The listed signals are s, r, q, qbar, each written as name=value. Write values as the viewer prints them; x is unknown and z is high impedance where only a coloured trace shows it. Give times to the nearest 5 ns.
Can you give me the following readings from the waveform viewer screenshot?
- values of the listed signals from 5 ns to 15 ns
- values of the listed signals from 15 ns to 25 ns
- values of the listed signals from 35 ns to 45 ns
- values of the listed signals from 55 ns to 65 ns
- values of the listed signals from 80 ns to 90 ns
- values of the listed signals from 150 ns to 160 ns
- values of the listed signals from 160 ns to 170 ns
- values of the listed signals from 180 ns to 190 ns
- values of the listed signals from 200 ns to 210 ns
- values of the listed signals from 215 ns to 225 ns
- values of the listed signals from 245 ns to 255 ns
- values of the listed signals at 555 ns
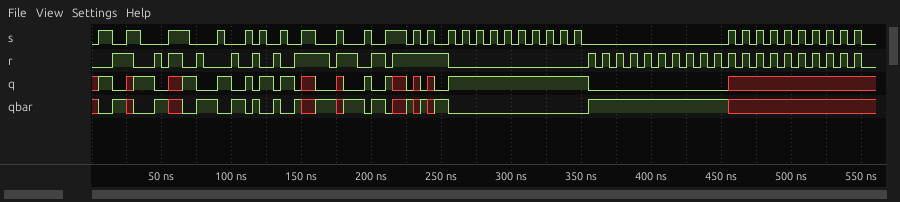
s=1, r=0, q=1, qbar=0
s=0, r=1, q=0, qbar=1
s=0, r=0, q=1, qbar=0
s=1, r=1, q=x, qbar=x
s=0, r=0, q=0, qbar=1
s=1, r=1, q=x, qbar=x
s=0, r=1, q=0, qbar=1
s=0, r=1, q=0, qbar=1
s=0, r=1, q=0, qbar=1
s=1, r=1, q=x, qbar=x
s=0, r=1, q=0, qbar=1
s=0, r=0, q=x, qbar=x
